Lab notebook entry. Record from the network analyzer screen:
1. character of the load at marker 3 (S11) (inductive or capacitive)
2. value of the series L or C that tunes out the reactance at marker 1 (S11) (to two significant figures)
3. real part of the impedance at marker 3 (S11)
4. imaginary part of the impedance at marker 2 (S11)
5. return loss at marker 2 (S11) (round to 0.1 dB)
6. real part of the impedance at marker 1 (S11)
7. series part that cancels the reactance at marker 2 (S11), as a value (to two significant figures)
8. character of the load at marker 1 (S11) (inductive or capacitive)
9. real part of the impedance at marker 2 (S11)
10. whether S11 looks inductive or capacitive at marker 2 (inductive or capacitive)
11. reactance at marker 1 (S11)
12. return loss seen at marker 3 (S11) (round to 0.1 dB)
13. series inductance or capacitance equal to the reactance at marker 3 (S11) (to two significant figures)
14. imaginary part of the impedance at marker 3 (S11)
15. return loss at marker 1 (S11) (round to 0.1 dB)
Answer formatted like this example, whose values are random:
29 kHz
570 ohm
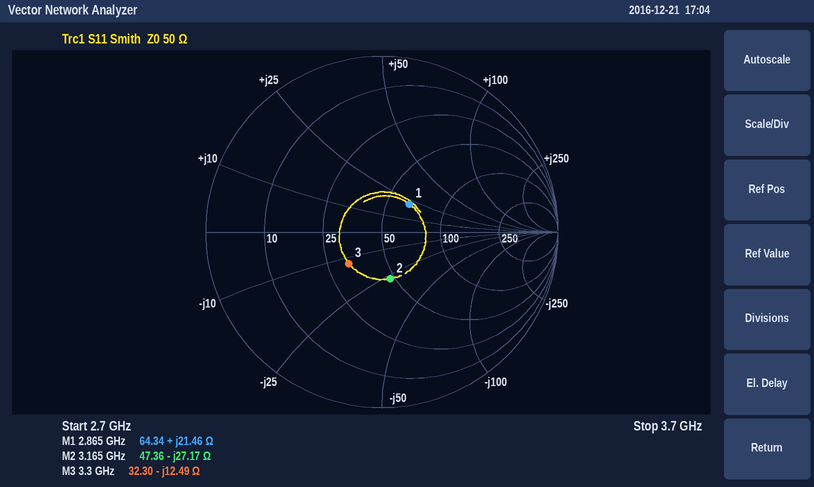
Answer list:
capacitive
2.6 pF
32.30 Ω
-27.17 Ω
11.4 dB
64.34 Ω
1.4 nH
inductive
47.36 Ω
capacitive
+21.46 Ω
11.7 dB
3.9 pF
-12.49 Ω
13.1 dB
